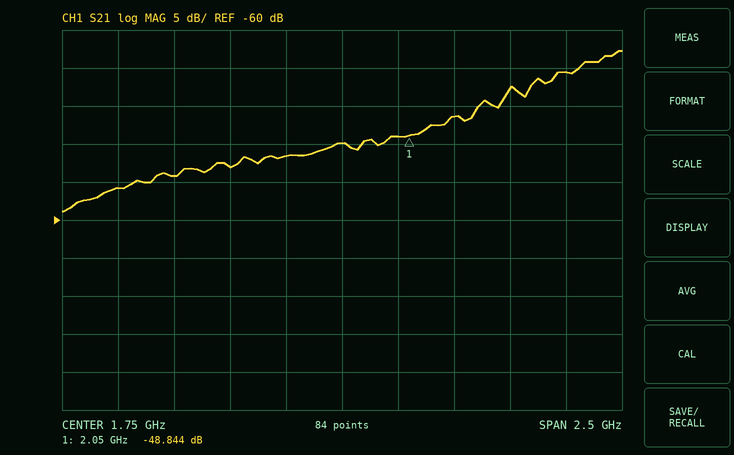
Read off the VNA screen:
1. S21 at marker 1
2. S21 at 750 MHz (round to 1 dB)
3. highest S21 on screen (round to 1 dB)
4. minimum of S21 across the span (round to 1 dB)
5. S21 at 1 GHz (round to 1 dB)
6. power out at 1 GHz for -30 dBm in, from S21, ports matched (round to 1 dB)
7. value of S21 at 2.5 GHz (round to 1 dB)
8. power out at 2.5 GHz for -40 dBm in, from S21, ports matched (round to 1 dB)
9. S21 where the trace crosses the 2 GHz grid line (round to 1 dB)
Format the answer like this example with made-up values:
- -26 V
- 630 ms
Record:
- -48.844 dB
- -56 dB
- -38 dB
- -59 dB
- -54 dB
- -84 dBm
- -43 dB
- -83 dBm
- -49 dB
